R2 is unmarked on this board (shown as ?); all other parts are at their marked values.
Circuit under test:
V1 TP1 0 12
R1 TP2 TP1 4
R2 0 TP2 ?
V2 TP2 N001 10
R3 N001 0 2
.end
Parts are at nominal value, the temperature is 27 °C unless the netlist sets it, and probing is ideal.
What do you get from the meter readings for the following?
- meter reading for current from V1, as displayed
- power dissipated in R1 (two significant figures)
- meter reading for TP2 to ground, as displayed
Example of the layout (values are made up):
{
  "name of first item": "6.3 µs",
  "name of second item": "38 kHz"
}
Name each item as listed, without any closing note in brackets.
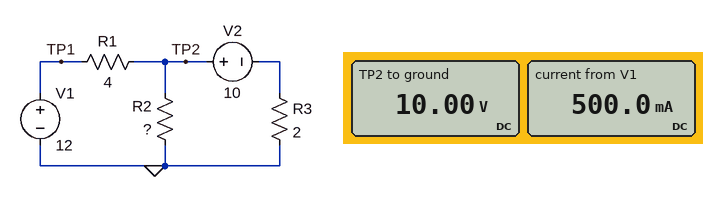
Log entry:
{
  "meter reading for current from V1, as displayed": "500.0 mA",
  "power dissipated in R1": "1.0 W",
  "meter reading for TP2 to ground, as displayed": "10.00 V"
}
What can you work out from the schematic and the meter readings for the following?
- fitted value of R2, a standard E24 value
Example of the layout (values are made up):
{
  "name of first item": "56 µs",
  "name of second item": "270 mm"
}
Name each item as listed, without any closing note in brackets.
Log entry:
{
  "fitted value of R2, a standard E24 value": "20 Ω"
}
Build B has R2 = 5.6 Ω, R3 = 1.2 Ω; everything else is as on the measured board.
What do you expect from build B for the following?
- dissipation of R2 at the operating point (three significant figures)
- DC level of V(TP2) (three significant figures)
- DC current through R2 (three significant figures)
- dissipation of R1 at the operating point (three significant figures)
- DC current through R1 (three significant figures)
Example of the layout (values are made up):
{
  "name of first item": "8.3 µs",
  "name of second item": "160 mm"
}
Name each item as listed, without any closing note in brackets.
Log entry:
{
  "dissipation of R2 at the operating point": "14.4 W",
  "DC level of V(TP2)": "8.98 V",
  "DC current through R2": "1.60 A",
  "dissipation of R1 at the operating point": "2.28 W",
  "DC current through R1": "755 mA"
}
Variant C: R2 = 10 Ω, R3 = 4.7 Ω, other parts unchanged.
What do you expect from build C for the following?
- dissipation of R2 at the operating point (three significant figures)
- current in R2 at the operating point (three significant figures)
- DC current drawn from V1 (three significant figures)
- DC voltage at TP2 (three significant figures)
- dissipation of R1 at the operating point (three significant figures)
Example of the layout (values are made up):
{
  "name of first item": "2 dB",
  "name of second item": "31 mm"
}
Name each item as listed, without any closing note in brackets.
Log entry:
{
  "dissipation of R2 at the operating point": "8.30 W",
  "current in R2 at the operating point": "911 mA",
  "DC current drawn from V1": "722 mA",
  "DC voltage at TP2": "9.11 V",
  "dissipation of R1 at the operating point": "2.09 W"
}
